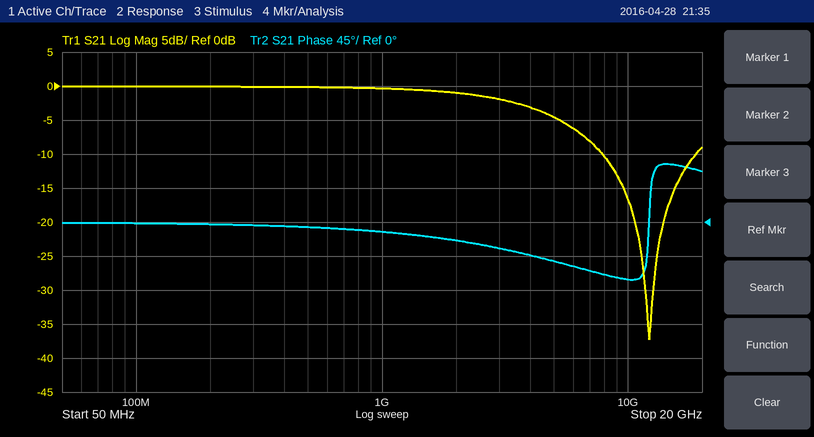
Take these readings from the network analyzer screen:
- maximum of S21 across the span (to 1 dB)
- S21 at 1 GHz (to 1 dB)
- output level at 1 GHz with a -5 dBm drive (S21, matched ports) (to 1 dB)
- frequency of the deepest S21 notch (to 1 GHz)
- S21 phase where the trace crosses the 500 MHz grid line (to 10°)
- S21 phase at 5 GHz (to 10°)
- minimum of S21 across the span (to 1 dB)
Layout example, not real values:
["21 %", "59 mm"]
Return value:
["0 dB", "0 dB", "-5 dBm", "12 GHz", "-10°", "-50°", "-37 dB"]
